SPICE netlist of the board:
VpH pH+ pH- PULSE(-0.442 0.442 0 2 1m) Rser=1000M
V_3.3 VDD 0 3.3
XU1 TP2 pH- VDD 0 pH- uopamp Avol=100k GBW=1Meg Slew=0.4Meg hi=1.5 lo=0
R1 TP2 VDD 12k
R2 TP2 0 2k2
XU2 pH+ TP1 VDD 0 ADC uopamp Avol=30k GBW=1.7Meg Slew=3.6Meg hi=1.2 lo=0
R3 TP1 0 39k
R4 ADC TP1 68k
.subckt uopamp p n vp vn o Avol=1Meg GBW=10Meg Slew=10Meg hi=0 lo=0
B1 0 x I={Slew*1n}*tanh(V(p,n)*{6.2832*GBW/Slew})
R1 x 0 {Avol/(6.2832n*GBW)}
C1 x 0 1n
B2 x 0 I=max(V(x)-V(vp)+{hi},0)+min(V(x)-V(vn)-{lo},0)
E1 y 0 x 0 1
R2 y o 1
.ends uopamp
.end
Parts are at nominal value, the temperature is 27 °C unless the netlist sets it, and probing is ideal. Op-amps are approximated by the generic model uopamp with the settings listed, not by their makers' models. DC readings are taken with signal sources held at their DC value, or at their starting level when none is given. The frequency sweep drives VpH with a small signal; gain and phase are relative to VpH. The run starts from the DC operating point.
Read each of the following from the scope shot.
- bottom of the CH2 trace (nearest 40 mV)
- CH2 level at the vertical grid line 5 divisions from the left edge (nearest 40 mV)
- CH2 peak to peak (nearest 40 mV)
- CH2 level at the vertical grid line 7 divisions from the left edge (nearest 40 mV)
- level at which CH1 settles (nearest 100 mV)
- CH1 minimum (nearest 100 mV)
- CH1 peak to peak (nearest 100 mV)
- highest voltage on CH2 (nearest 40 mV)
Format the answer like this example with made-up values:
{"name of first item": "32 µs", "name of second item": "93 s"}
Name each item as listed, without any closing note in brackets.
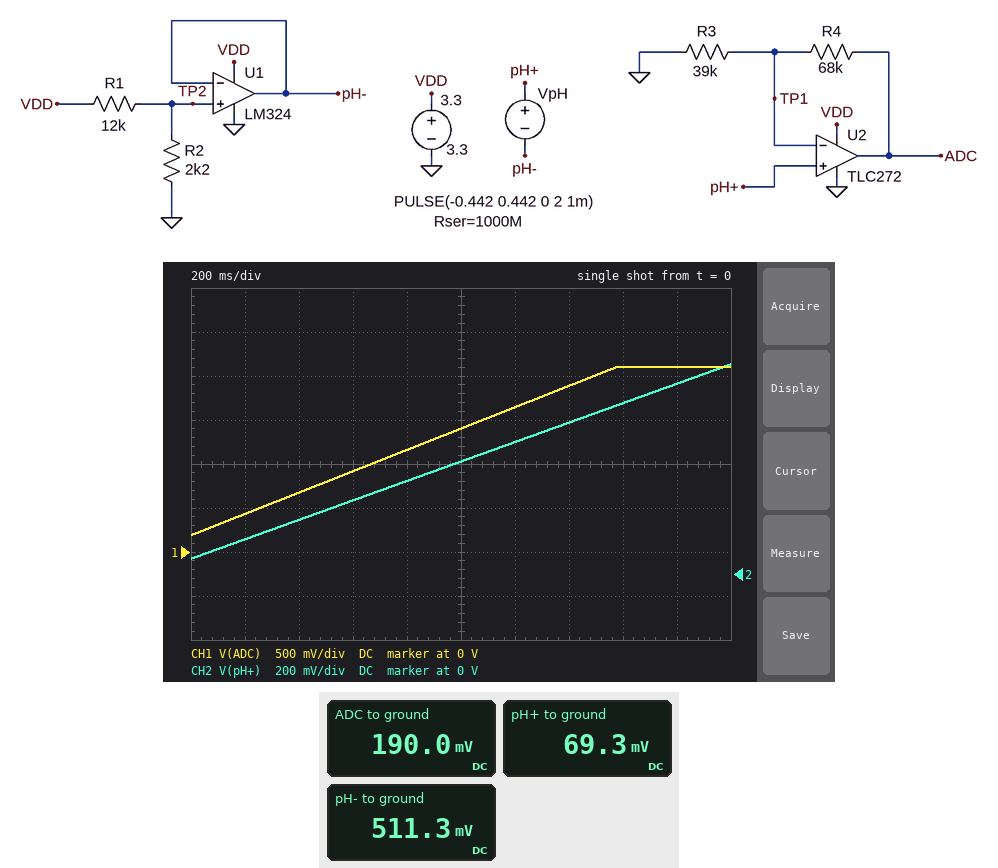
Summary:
{"bottom of the CH2 trace": "80 mV", "CH2 level at the vertical grid line 5 divisions from the left edge": "520 mV", "CH2 peak to peak": "880 mV", "CH2 level at the vertical grid line 7 divisions from the left edge": "680 mV", "level at which CH1 settles": "2.1 V", "CH1 minimum": "200 mV", "CH1 peak to peak": "1.9 V", "highest voltage on CH2": "960 mV"}
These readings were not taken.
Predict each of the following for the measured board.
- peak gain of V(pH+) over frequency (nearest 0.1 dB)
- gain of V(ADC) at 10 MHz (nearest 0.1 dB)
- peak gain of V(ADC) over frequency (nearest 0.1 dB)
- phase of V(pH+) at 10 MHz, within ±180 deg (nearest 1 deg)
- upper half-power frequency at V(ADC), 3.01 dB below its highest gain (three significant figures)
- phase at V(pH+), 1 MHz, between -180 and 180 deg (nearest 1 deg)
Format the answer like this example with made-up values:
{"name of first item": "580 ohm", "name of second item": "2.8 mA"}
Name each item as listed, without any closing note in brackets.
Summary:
{"peak gain of V(pH+) over frequency": "0 dB", "gain of V(ADC) at 10 MHz": "-15.4 dB", "peak gain of V(ADC) over frequency": "8.8 dB", "phase of V(pH+) at 10 MHz, within ±180 deg": "0 deg", "upper half-power frequency at V(ADC), 3.01 dB below its highest gain": "620 kHz", "phase at V(pH+), 1 MHz, between -180 and 180 deg": "0 deg"}
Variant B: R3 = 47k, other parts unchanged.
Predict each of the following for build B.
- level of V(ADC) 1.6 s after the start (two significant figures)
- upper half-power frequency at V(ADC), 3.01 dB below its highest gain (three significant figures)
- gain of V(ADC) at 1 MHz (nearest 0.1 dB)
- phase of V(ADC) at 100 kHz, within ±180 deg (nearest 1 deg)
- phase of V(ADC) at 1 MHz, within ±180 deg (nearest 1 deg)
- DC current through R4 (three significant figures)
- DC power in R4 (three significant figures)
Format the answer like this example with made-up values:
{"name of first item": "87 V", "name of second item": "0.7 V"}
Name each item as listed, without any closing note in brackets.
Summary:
{"level of V(ADC) 1.6 s after the start": "1.9 V", "upper half-power frequency at V(ADC), 3.01 dB below its highest gain": "695 kHz", "gain of V(ADC) at 1 MHz": "2.9 dB", "phase of V(ADC) at 100 kHz, within ±180 deg": "-8 deg", "phase of V(ADC) at 1 MHz, within ±180 deg": "-55 deg", "DC current through R4": "1.47 µA", "DC power in R4": "148 nW"}
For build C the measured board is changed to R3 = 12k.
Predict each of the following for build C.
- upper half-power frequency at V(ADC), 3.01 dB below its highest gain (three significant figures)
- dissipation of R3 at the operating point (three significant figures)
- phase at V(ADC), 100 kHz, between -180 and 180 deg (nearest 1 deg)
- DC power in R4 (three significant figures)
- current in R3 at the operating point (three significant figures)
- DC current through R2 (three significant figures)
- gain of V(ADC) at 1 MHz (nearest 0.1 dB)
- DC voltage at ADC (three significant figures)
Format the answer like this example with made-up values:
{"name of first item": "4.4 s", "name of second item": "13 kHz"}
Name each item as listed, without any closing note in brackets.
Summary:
{"upper half-power frequency at V(ADC), 3.01 dB below its highest gain": "255 kHz", "dissipation of R3 at the operating point": "400 nW", "phase at V(ADC), 100 kHz, between -180 and 180 deg": "-21 deg", "DC power in R4": "2.26 µW", "current in R3 at the operating point": "5.77 µA", "DC current through R2": "232 µA", "gain of V(ADC) at 1 MHz": "4.3 dB", "DC voltage at ADC": "462 mV"}
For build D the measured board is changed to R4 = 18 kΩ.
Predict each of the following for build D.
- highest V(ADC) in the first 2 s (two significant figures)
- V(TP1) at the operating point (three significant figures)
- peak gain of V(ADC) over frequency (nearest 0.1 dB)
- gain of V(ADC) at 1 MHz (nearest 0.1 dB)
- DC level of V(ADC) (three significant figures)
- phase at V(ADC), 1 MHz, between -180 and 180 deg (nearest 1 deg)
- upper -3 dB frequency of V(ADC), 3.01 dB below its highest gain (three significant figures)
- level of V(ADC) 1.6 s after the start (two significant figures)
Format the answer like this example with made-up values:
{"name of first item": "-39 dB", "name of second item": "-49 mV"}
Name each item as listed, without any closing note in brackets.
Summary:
{"highest V(ADC) in the first 2 s": "1.4 V", "V(TP1) at the operating point": "69.3 mV", "peak gain of V(ADC) over frequency": "3.3 dB", "gain of V(ADC) at 1 MHz": "0.9 dB", "DC level of V(ADC)": "101 mV", "phase at V(ADC), 1 MHz, between -180 and 180 deg": "-41 deg", "upper -3 dB frequency of V(ADC), 3.01 dB below its highest gain": "1.16 MHz", "level of V(ADC) 1.6 s after the start": "1.1 V"}
